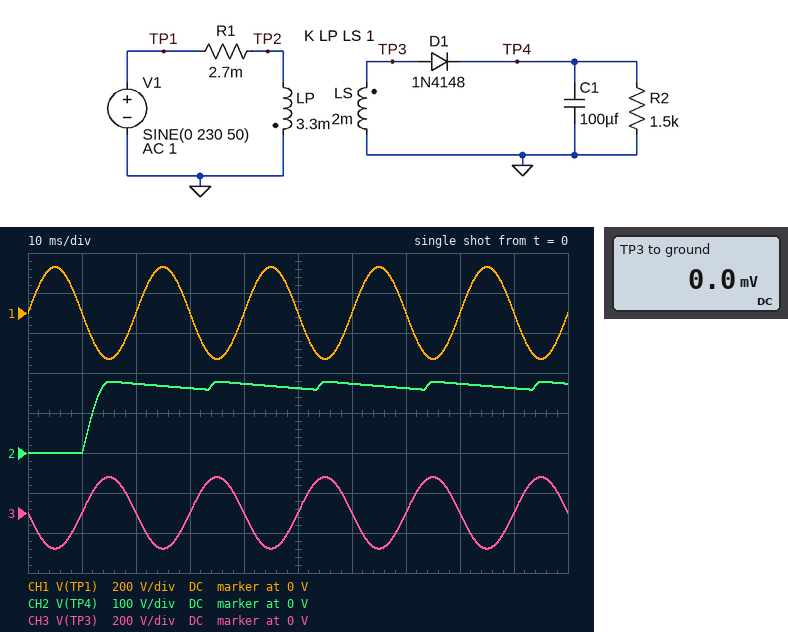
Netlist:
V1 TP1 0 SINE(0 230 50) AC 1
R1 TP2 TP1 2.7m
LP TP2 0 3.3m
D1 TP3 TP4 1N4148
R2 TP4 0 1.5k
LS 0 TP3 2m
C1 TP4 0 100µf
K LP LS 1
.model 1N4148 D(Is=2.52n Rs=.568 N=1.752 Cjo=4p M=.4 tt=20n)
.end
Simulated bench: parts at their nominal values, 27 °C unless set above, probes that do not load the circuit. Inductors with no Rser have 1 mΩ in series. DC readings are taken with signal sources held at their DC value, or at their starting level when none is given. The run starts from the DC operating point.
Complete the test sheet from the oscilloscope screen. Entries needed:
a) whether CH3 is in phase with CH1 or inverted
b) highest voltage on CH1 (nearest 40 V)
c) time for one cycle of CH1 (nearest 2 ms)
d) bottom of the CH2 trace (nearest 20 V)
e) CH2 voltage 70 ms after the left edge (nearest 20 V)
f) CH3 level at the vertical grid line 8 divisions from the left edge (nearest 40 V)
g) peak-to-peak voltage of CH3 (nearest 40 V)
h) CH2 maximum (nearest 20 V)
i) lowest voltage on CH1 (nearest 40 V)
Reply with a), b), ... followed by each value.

a) inverted
b) 240 V
c) 20 ms
d) 0 V
e) 160 V
f) 0 V
g) 360 V
h) 180 V
i) -240 V
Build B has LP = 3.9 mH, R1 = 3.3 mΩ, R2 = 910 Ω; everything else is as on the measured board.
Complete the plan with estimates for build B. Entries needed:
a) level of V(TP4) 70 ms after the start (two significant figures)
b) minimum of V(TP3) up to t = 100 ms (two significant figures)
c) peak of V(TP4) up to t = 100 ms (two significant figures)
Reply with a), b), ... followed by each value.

a) 140 V
b) -160 V
c) 160 V
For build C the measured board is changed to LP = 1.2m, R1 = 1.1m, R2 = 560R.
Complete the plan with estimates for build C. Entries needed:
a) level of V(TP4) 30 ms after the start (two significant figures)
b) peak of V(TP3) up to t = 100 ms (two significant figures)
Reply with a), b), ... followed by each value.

a) 230 V
b) 300 V
